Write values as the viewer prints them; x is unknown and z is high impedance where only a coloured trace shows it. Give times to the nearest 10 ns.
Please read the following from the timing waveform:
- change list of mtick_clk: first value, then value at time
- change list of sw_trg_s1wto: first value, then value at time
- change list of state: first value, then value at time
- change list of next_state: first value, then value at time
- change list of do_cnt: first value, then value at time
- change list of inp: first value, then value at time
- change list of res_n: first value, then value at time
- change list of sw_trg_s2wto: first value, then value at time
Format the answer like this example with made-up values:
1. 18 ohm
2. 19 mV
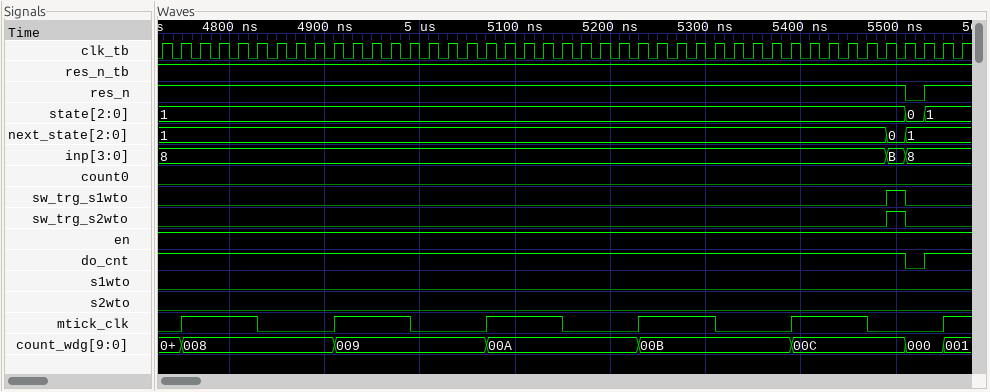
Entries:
1. 0, 1 at 4750 ns, 0 at 4830 ns, 1 at 4910 ns, 0 at 4990 ns, 1 at 5070 ns, 0 at 5150 ns, 1 at 5230 ns, 0 at 5310 ns, 1 at 5390 ns, 0 at 5470 ns, 1 at 5550 ns
2. 0, 1 at 5490 ns, 0 at 5510 ns
3. 1, 0 at 5510 ns, 1 at 5530 ns
4. 1, 0 at 5490 ns, 1 at 5510 ns
5. 1, 0 at 5510 ns, 1 at 5530 ns
6. 8, B at 5490 ns, 8 at 5510 ns
7. 1, 0 at 5510 ns, 1 at 5530 ns
8. 0, 1 at 5490 ns, 0 at 5510 ns
